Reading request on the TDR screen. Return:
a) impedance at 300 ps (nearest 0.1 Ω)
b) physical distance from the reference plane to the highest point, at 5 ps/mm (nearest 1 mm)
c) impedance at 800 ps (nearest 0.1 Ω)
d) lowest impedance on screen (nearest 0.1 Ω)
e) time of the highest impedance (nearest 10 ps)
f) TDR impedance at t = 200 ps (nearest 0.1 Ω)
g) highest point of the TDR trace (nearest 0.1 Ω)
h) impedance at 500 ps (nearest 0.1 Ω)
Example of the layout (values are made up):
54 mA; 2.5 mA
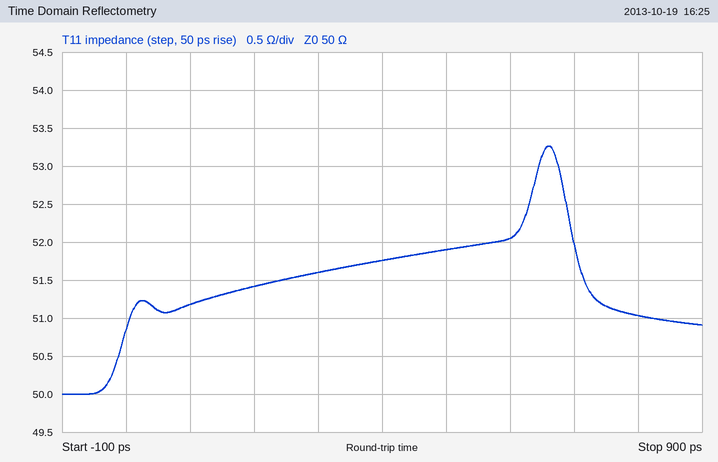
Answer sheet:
51.6 Ω; 66 mm; 51.0 Ω; 50.0 Ω; 660 ps; 51.4 Ω; 53.3 Ω; 51.9 Ω
